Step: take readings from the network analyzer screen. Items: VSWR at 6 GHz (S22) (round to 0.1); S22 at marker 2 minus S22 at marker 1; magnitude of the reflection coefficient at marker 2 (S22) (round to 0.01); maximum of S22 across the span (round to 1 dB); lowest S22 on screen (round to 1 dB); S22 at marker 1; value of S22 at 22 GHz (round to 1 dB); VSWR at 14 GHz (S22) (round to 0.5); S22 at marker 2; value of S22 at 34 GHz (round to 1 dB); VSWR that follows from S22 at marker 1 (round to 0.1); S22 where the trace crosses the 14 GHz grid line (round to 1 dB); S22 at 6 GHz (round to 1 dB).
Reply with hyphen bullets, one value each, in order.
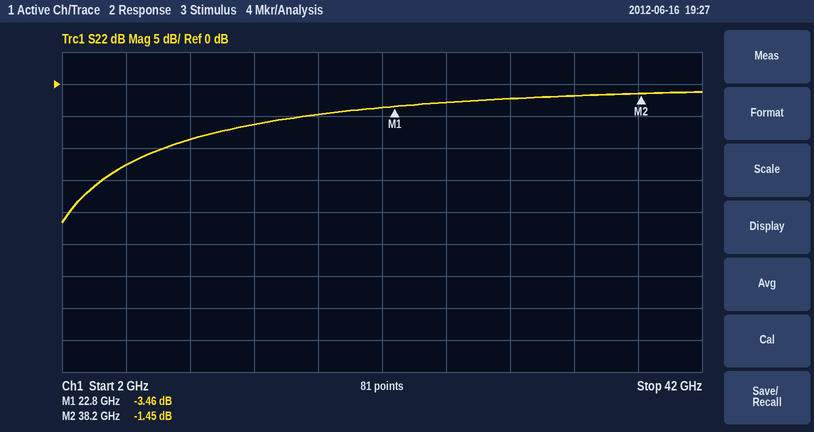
- 1.6
- 2.01 dB
- 0.85
- -1 dB
- -22 dB
- -3.46 dB
- -4 dB
- 3.0
- -1.45 dB
- -2 dB
- 5.1
- -6 dB
- -13 dB
